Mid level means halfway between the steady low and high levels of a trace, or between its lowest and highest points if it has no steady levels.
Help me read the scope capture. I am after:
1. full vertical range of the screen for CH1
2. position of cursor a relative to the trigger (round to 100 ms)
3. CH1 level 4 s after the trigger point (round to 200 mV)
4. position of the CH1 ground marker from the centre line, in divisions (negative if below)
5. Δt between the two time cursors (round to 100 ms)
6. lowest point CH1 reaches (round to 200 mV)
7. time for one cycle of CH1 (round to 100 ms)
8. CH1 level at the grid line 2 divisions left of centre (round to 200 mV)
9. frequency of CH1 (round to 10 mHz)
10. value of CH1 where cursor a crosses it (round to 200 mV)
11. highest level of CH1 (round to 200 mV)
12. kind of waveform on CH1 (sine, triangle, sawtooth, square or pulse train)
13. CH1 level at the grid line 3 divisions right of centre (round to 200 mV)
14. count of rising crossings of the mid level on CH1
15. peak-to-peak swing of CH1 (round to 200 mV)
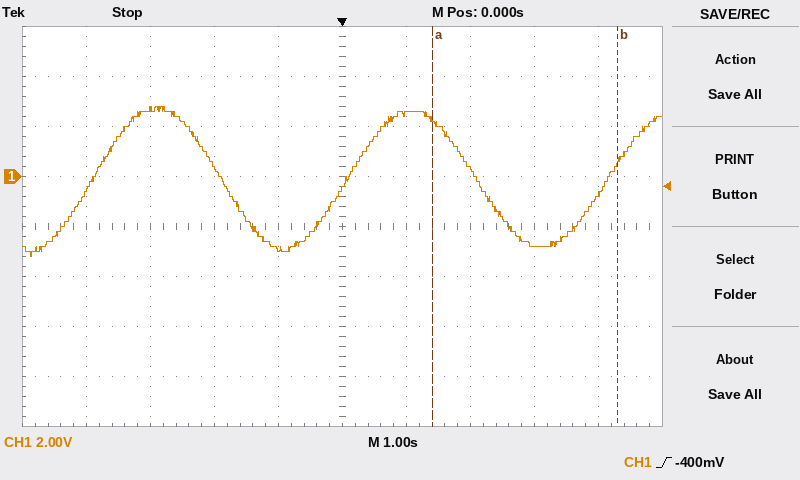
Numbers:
16 V
+1.4 s
-800 mV
+1.0 div
2.9 s
-3.2 V
4.0 s
400 mV
250 mHz
2.2 V
2.8 V
sine
-2.8 V
3
6.0 V
